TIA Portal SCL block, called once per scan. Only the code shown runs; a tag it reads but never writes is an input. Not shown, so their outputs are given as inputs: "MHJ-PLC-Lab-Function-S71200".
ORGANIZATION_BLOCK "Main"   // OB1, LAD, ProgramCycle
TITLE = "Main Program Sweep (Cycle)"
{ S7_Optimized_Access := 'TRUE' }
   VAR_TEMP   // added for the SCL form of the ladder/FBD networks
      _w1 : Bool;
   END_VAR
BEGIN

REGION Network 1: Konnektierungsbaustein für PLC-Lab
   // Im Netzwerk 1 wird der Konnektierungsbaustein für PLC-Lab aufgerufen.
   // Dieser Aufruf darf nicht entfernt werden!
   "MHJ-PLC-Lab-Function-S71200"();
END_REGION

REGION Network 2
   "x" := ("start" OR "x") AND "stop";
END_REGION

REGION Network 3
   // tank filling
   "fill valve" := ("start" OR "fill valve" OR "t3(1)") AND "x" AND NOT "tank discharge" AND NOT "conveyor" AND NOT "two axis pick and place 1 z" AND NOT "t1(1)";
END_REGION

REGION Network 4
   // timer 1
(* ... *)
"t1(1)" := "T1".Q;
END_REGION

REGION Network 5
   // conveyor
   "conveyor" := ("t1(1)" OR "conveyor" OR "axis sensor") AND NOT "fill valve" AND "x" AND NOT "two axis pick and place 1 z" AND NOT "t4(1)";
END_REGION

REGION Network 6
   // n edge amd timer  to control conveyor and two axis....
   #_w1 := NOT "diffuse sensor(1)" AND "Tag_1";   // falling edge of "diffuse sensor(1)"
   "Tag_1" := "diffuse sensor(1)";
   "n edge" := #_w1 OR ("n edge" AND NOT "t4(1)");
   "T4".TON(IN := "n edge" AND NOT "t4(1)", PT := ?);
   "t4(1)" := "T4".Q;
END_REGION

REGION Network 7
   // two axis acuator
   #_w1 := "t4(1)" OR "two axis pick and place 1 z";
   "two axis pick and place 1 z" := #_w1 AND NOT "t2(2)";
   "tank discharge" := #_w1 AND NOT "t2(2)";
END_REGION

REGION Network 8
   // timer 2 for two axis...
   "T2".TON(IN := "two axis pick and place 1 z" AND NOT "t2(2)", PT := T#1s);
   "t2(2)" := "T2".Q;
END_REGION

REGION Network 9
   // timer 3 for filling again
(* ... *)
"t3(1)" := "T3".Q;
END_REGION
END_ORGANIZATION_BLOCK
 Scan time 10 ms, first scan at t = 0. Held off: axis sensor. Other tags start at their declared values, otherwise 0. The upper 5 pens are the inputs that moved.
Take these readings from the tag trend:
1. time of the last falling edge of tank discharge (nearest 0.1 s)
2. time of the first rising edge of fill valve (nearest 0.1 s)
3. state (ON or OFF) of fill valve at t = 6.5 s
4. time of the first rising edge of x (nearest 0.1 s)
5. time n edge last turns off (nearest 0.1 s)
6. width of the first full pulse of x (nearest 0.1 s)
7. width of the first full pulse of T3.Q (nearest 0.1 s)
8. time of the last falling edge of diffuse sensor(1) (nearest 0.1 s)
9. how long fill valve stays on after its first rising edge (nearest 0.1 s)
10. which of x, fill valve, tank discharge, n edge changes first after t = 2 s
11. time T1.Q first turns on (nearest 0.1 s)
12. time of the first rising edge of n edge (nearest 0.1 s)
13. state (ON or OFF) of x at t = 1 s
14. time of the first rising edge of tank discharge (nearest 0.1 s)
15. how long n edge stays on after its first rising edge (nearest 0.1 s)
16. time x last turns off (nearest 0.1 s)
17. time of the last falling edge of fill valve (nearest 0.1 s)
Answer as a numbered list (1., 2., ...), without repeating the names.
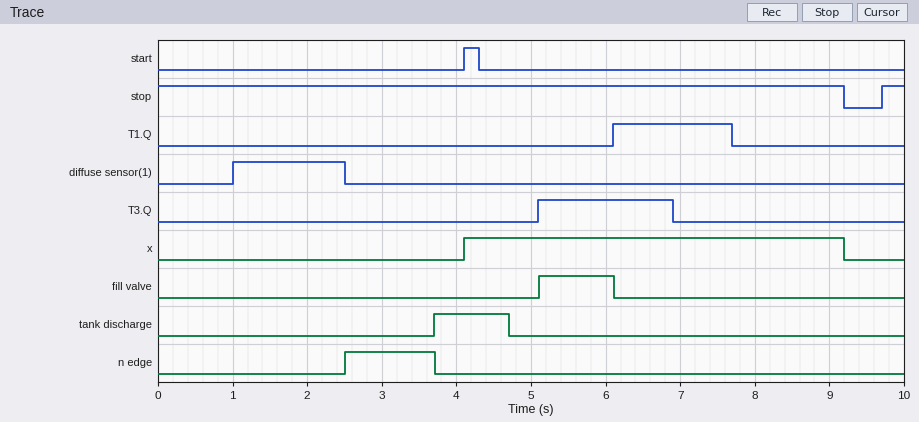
1. 4.7 s
2. 5.1 s
3. OFF
4. 4.1 s
5. 3.7 s
6. 5.1 s
7. 1.8 s
8. 2.5 s
9. 1.0 s
10. n edge
11. 6.1 s
12. 2.5 s
13. OFF
14. 3.7 s
15. 1.2 s
16. 9.2 s
17. 6.1 s
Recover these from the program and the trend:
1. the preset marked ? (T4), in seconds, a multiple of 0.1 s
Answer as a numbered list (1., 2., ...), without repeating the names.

1. 1.2 s
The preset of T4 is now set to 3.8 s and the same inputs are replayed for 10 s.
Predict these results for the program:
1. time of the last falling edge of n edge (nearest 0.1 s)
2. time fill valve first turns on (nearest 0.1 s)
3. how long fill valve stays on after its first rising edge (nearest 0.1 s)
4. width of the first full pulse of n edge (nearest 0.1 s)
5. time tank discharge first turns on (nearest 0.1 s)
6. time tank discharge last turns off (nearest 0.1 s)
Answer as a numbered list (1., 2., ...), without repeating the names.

1. 6.3 s
2. 4.1 s
3. 2.0 s
4. 3.8 s
5. 6.3 s
6. 7.3 s
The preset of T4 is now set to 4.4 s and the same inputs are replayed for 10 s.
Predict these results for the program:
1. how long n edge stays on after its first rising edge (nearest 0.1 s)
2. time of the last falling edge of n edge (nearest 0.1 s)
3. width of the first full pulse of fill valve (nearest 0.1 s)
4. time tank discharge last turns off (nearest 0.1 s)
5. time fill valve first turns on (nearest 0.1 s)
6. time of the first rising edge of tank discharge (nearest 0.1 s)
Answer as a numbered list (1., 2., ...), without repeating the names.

1. 4.4 s
2. 6.9 s
3. 2.0 s
4. 7.9 s
5. 4.1 s
6. 6.9 s
